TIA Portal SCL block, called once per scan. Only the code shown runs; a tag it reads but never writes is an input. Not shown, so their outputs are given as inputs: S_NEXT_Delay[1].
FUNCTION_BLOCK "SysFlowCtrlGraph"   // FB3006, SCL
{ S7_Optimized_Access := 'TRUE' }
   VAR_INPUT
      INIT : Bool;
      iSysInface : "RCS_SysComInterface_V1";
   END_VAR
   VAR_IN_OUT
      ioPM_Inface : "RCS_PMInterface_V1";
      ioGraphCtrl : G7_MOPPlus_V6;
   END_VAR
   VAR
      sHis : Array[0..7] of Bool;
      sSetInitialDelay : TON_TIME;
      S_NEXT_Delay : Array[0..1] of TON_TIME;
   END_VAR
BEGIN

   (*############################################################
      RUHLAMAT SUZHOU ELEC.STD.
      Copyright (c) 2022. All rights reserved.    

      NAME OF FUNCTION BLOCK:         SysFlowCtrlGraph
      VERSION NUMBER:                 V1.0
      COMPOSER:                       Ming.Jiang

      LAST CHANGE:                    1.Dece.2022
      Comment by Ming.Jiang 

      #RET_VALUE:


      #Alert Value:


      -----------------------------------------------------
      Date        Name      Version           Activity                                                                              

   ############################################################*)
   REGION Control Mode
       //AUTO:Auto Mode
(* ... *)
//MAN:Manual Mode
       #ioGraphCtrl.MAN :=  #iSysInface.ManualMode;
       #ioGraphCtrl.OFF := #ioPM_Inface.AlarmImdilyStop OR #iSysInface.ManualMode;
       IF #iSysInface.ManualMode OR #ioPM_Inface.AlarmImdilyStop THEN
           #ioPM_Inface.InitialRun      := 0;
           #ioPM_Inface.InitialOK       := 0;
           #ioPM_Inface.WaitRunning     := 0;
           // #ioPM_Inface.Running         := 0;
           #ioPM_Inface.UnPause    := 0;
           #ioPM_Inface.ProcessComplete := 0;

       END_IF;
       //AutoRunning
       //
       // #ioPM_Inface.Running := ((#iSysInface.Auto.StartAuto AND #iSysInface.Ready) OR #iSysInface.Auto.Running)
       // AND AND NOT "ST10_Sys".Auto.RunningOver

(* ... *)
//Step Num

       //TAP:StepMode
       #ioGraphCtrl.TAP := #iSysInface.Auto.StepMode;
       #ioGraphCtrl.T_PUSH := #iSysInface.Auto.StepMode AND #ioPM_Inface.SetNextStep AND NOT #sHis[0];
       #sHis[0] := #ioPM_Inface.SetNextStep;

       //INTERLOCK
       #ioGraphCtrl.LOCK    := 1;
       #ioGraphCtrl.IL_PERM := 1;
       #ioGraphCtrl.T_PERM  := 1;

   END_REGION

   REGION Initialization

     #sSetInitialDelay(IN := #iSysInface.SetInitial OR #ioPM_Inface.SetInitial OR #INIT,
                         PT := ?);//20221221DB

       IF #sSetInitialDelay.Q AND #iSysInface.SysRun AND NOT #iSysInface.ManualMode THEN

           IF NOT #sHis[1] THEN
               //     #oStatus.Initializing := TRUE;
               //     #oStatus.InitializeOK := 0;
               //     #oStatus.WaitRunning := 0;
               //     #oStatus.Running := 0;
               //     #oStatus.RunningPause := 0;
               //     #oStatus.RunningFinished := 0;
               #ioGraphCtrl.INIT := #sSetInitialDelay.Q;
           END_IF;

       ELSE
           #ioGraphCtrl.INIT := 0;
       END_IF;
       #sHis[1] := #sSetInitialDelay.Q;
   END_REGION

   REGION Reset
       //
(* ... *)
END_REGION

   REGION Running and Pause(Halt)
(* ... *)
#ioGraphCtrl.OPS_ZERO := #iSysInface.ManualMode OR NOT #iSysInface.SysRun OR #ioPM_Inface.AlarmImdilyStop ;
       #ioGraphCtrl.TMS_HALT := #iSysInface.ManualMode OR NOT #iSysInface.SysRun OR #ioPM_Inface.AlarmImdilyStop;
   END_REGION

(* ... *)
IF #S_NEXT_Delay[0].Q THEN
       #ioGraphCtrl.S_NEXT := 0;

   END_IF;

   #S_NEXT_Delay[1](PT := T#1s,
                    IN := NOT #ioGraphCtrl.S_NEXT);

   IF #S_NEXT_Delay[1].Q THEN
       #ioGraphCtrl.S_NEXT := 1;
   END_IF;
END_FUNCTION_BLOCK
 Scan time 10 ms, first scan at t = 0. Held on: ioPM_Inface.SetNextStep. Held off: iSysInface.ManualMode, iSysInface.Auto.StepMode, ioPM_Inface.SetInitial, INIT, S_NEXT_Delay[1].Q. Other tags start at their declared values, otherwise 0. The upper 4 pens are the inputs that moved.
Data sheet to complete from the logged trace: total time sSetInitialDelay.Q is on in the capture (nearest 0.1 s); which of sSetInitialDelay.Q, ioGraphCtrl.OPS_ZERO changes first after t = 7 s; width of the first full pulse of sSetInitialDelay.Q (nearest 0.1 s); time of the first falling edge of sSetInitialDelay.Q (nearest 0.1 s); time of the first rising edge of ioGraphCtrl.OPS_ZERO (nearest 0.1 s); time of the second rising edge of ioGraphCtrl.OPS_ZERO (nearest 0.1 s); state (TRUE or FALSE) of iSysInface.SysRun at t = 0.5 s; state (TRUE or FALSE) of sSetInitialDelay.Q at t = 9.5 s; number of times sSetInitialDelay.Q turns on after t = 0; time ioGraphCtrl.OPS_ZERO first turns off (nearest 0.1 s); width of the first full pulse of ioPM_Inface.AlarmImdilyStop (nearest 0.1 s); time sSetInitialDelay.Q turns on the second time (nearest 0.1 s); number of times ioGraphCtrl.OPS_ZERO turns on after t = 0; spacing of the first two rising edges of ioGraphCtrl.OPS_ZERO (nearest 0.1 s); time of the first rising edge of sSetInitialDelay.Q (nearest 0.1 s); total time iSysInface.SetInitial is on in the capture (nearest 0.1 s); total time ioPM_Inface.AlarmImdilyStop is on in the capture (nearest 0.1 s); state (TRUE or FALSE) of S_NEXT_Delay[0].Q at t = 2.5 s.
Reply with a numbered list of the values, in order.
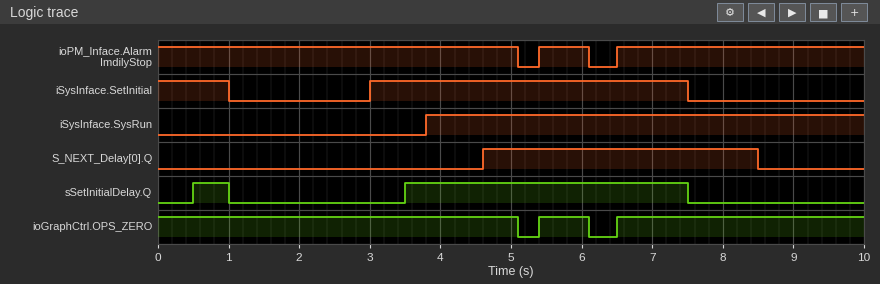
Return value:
1. 4.5 s
2. sSetInitialDelay.Q
3. 0.5 s
4. 1.0 s
5. 5.4 s
6. 6.5 s
7. FALSE
8. FALSE
9. 2
10. 5.1 s
11. 0.7 s
12. 3.5 s
13. 2
14. 1.1 s
15. 0.5 s
16. 5.5 s
17. 9.3 s
18. FALSE
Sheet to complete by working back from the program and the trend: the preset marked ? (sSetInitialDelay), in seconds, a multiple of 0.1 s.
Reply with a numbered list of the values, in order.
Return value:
1. 0.5 s
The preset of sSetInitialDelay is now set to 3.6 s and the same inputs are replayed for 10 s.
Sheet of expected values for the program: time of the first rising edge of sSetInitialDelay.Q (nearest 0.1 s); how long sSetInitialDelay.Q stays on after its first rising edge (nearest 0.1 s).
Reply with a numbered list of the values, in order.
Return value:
1. 6.6 s
2. 0.9 s
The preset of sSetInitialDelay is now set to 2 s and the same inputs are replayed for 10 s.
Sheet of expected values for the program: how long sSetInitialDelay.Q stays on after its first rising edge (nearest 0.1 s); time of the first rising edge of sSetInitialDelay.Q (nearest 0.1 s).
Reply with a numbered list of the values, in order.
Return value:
1. 2.5 s
2. 5.0 s
